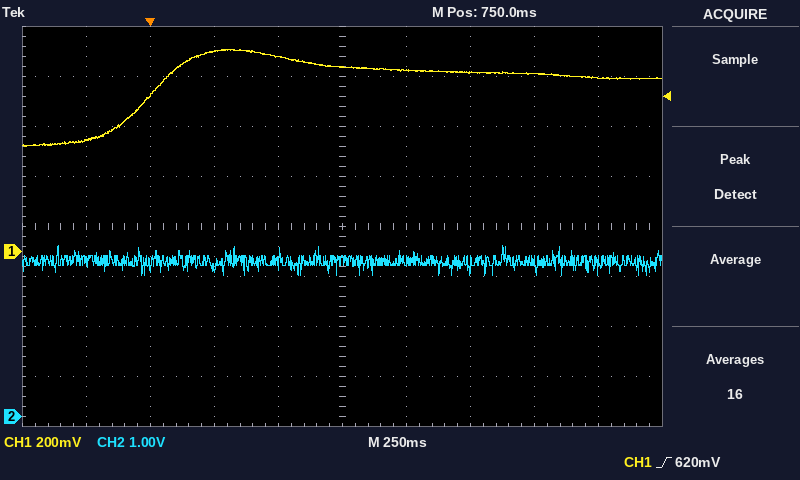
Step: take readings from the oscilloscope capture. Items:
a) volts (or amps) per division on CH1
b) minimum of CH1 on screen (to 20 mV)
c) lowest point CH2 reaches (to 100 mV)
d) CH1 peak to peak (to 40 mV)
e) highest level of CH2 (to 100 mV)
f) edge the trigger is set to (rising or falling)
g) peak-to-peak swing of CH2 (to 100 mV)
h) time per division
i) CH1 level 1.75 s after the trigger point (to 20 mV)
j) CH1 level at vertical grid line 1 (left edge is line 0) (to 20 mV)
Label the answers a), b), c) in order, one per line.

a) 200 mV
b) 420 mV
c) 2.8 V
d) 400 mV
e) 3.4 V
f) rising
g) 600 mV
h) 250 ms
i) 700 mV
j) 440 mV
